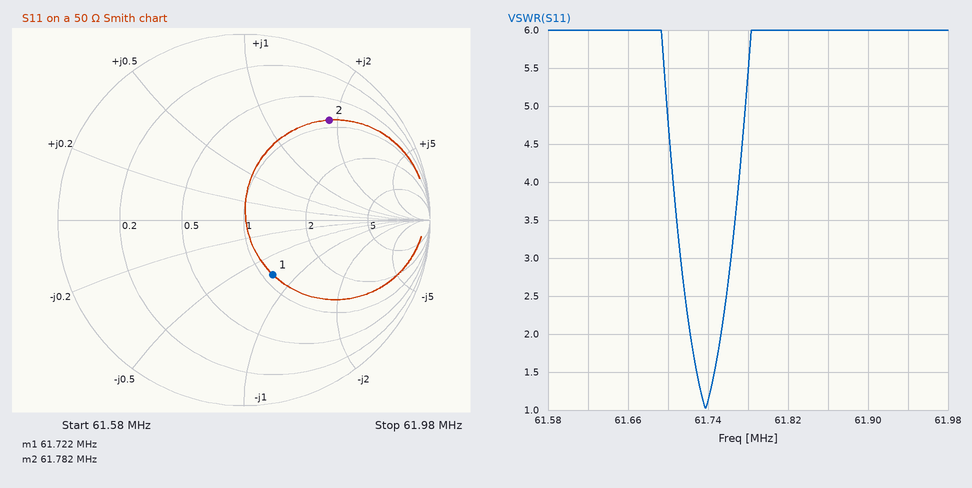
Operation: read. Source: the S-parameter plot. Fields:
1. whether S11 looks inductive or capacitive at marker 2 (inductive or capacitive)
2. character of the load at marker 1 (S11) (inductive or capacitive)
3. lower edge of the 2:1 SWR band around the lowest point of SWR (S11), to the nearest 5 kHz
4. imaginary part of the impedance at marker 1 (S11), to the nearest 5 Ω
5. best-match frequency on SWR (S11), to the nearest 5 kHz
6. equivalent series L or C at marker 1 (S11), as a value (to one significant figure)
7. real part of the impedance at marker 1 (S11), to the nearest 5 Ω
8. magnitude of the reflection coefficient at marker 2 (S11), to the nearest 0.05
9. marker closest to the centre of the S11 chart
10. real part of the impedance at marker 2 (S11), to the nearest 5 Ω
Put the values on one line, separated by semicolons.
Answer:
inductive; capacitive; 61.720 MHz; -35 Ω; 61.735 MHz; 70 pF; 55 Ω; 0.70; marker 1; 45 Ω
